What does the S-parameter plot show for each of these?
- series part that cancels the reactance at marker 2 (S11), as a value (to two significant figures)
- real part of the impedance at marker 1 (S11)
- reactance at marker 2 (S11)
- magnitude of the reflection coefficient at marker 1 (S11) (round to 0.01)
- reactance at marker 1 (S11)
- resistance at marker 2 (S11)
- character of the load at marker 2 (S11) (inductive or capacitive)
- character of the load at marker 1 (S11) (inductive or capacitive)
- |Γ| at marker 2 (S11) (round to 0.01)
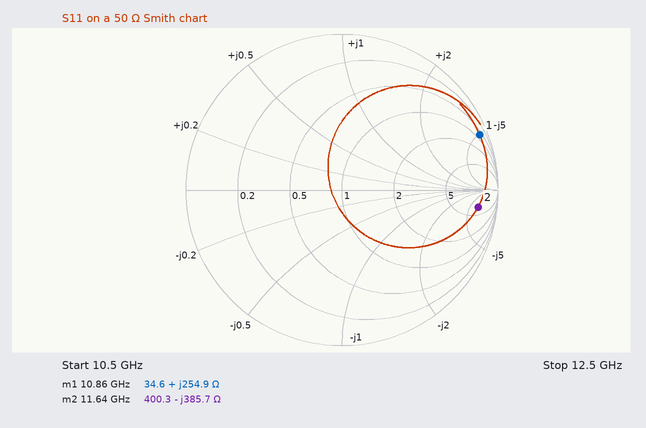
5.3 nH
34.6 Ω
-385.7 Ω
0.95
+254.9 Ω
400.3 Ω
capacitive
inductive
0.88
